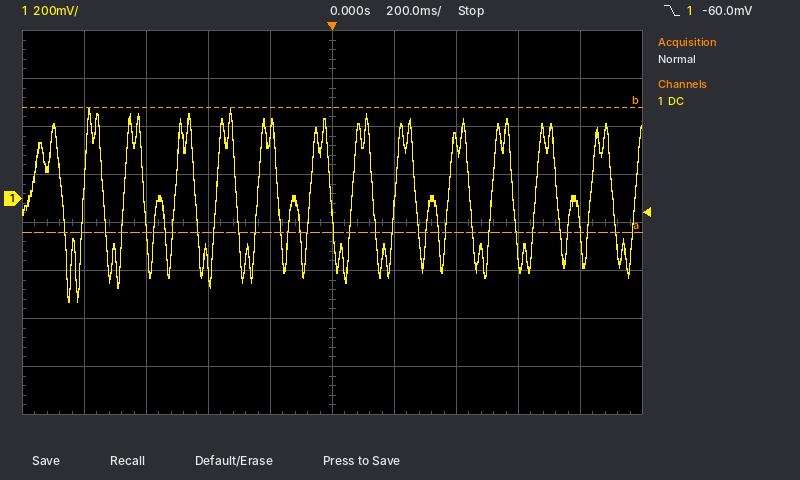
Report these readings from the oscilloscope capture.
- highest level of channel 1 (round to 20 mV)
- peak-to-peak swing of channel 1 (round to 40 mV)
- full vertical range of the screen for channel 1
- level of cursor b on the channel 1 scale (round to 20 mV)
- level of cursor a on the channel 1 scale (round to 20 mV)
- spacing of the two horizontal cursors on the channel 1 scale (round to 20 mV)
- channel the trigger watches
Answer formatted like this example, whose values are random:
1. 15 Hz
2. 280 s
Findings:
1. 380 mV
2. 800 mV
3. 1.6 V
4. 380 mV
5. -140 mV
6. 520 mV
7. channel 1
